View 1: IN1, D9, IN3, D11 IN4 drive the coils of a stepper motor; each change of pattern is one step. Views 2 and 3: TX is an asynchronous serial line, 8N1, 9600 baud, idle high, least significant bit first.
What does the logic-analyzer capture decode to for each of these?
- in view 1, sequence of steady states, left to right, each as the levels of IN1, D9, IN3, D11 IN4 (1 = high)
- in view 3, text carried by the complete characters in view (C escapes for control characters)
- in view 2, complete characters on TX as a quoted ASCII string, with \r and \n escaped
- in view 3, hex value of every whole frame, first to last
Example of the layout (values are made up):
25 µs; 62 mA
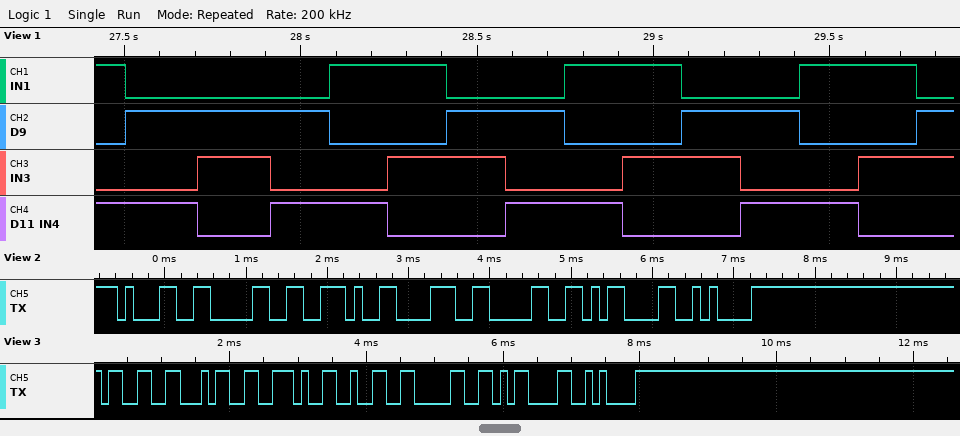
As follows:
1001 0101 0110 0101 1001 1010 0110 0101 1001 1010 0110 0101 1001 1010 0110; "34.20\r\n"; "10.80\r\n"; 33 34 2E 32 30 0D 0A
